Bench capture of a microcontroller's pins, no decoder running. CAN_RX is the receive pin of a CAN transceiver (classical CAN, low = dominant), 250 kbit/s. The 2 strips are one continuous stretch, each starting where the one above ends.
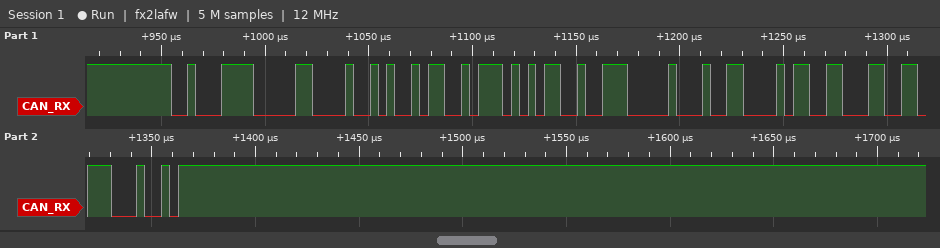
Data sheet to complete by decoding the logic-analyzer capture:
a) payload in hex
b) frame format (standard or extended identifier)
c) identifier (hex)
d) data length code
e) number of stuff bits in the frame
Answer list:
4A 59 75 64 E0 13 0B 31
standard
0x23C
8
2
